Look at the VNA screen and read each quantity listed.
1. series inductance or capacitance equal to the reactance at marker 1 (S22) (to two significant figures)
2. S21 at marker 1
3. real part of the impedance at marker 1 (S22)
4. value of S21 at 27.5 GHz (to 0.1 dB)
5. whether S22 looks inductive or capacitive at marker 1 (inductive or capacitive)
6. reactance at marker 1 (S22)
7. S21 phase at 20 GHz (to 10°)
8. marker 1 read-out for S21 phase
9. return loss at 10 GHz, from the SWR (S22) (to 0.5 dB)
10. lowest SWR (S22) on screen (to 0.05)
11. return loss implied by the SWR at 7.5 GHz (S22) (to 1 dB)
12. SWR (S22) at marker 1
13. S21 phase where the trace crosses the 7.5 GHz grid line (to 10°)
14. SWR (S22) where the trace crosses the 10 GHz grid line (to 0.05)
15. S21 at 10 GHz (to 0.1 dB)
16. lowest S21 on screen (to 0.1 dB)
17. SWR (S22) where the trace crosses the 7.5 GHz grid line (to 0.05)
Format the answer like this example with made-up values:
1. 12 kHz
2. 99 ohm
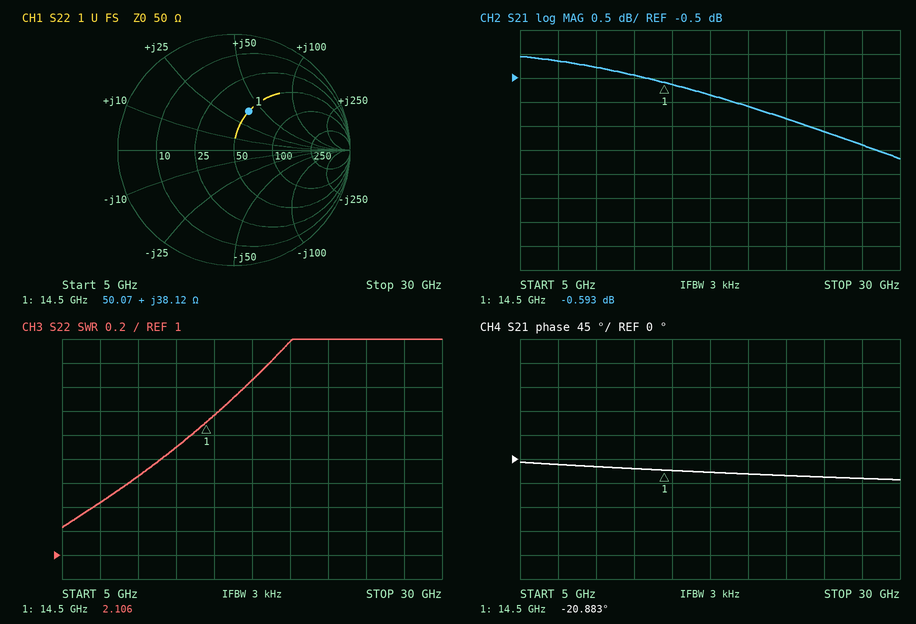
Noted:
1. 420 pH
2. -0.593 dB
3. 50.07 Ω
4. -1.9 dB
5. inductive
6. +38.12 Ω
7. -30°
8. -20.883°
9. 12.0 dB
10. 1.25
11. 15 dB
12. 2.106
13. -10°
14. 1.65
15. -0.3 dB
16. -2.2 dB
17. 1.45
